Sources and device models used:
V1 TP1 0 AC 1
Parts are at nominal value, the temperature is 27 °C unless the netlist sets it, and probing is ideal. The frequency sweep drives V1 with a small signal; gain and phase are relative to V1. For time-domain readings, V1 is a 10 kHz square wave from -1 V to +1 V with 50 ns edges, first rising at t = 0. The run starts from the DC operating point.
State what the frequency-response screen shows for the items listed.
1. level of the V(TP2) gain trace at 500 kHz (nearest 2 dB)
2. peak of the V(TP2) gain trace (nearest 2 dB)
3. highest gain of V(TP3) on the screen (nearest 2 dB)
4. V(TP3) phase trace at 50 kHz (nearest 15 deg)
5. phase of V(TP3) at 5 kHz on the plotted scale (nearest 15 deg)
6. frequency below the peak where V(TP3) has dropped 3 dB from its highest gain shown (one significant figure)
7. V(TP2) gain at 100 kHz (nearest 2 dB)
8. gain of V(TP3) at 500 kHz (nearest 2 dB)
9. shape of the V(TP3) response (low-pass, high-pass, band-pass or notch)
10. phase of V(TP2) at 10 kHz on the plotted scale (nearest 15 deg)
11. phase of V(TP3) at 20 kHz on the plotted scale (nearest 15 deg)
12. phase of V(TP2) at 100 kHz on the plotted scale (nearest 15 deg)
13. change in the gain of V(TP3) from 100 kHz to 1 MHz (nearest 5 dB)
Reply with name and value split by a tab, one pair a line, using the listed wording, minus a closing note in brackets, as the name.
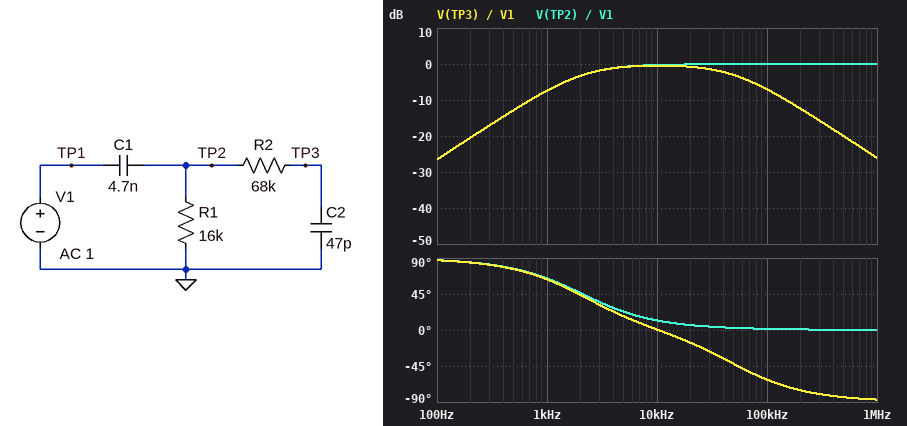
level of the V(TP2) gain trace at 500 kHz	0 dB
peak of the V(TP2) gain trace	0 dB
highest gain of V(TP3) on the screen	0 dB
V(TP3) phase trace at 50 kHz	-45 deg
phase of V(TP3) at 5 kHz on the plotted scale	15 deg
frequency below the peak where V(TP3) has dropped 3 dB from its highest gain shown	2 kHz
V(TP2) gain at 100 kHz	0 dB
gain of V(TP3) at 500 kHz	-20 dB
shape of the V(TP3) response	band-pass
phase of V(TP2) at 10 kHz on the plotted scale	15 deg
phase of V(TP3) at 20 kHz on the plotted scale	-15 deg
phase of V(TP2) at 100 kHz on the plotted scale	0 deg
change in the gain of V(TP3) from 100 kHz to 1 MHz	-20 dB
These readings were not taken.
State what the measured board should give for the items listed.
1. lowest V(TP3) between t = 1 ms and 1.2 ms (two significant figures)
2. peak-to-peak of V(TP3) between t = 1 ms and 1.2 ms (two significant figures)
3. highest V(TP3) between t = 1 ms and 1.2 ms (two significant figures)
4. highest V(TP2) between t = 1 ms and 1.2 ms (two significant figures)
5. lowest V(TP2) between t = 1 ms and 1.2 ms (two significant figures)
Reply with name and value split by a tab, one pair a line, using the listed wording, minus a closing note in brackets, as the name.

lowest V(TP3) between t = 1 ms and 1.2 ms	-1.1 V
peak-to-peak of V(TP3) between t = 1 ms and 1.2 ms	2.2 V
highest V(TP3) between t = 1 ms and 1.2 ms	1.1 V
highest V(TP2) between t = 1 ms and 1.2 ms	1.3 V
lowest V(TP2) between t = 1 ms and 1.2 ms	-1.3 V
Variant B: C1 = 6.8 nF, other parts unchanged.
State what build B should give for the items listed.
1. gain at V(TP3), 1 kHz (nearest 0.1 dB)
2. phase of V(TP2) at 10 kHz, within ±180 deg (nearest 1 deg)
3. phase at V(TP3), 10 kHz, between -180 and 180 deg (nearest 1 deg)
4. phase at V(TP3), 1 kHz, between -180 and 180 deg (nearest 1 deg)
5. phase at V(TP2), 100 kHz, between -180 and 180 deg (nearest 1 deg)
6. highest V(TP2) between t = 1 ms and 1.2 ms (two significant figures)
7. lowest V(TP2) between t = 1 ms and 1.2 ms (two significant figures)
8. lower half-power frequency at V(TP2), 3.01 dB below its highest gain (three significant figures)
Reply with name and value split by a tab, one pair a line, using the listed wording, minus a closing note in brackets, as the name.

gain at V(TP3), 1 kHz	-5.0 dB
phase of V(TP2) at 10 kHz, within ±180 deg	8 deg
phase at V(TP3), 10 kHz, between -180 and 180 deg	-3 deg
phase at V(TP3), 1 kHz, between -180 and 180 deg	54 deg
phase at V(TP2), 100 kHz, between -180 and 180 deg	1 deg
highest V(TP2) between t = 1 ms and 1.2 ms	1.2 V
lowest V(TP2) between t = 1 ms and 1.2 ms	-1.2 V
lower half-power frequency at V(TP2), 3.01 dB below its highest gain	1.47 kHz
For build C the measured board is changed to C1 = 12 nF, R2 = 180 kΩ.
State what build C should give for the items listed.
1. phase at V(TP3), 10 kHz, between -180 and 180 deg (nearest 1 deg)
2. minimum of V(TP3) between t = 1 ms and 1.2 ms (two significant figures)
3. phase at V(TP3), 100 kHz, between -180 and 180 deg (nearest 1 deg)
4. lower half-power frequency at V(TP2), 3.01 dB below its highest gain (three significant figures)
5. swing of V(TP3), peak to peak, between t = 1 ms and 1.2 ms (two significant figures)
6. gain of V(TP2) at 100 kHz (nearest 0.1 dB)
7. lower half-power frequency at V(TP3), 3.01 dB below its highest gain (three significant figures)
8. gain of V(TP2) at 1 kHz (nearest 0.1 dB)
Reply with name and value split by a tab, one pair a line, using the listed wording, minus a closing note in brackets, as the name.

phase at V(TP3), 10 kHz, between -180 and 180 deg	-23 deg
minimum of V(TP3) between t = 1 ms and 1.2 ms	-950 mV
phase at V(TP3), 100 kHz, between -180 and 180 deg	-79 deg
lower half-power frequency at V(TP2), 3.01 dB below its highest gain	832 Hz
swing of V(TP3), peak to peak, between t = 1 ms and 1.2 ms	1.9 V
gain of V(TP2) at 100 kHz	0 dB
lower half-power frequency at V(TP3), 3.01 dB below its highest gain	762 Hz
gain of V(TP2) at 1 kHz	-2.3 dB
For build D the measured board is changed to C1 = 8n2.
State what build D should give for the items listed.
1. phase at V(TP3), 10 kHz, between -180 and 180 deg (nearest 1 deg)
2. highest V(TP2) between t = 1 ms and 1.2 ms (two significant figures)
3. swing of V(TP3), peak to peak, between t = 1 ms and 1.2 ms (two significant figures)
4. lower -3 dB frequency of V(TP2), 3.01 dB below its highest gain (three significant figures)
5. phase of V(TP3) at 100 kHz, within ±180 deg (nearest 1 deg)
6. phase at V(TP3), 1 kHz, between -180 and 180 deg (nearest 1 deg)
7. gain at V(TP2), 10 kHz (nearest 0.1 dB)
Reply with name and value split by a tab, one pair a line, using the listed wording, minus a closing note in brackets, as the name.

phase at V(TP3), 10 kHz, between -180 and 180 deg	-4 deg
highest V(TP2) between t = 1 ms and 1.2 ms	1.2 V
swing of V(TP3), peak to peak, between t = 1 ms and 1.2 ms	2.1 V
lower -3 dB frequency of V(TP2), 3.01 dB below its highest gain	1.22 kHz
phase of V(TP3) at 100 kHz, within ±180 deg	-63 deg
phase at V(TP3), 1 kHz, between -180 and 180 deg	49 deg
gain at V(TP2), 10 kHz	-0.1 dB
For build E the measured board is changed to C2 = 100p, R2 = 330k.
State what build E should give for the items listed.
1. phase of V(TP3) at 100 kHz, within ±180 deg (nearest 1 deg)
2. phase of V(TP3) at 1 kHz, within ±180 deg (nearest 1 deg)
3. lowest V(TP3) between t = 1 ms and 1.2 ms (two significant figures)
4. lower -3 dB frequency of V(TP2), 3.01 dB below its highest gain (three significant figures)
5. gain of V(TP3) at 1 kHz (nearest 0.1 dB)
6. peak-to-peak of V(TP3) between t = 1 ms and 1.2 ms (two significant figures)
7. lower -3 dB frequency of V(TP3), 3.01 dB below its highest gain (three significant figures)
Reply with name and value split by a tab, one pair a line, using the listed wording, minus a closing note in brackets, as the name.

phase of V(TP3) at 100 kHz, within ±180 deg	-86 deg
phase of V(TP3) at 1 kHz, within ±180 deg	53 deg
lowest V(TP3) between t = 1 ms and 1.2 ms	-560 mV
lower -3 dB frequency of V(TP2), 3.01 dB below its highest gain	2.17 kHz
gain of V(TP3) at 1 kHz	-7.6 dB
peak-to-peak of V(TP3) between t = 1 ms and 1.2 ms	1.1 V
lower -3 dB frequency of V(TP3), 3.01 dB below its highest gain	1.23 kHz
